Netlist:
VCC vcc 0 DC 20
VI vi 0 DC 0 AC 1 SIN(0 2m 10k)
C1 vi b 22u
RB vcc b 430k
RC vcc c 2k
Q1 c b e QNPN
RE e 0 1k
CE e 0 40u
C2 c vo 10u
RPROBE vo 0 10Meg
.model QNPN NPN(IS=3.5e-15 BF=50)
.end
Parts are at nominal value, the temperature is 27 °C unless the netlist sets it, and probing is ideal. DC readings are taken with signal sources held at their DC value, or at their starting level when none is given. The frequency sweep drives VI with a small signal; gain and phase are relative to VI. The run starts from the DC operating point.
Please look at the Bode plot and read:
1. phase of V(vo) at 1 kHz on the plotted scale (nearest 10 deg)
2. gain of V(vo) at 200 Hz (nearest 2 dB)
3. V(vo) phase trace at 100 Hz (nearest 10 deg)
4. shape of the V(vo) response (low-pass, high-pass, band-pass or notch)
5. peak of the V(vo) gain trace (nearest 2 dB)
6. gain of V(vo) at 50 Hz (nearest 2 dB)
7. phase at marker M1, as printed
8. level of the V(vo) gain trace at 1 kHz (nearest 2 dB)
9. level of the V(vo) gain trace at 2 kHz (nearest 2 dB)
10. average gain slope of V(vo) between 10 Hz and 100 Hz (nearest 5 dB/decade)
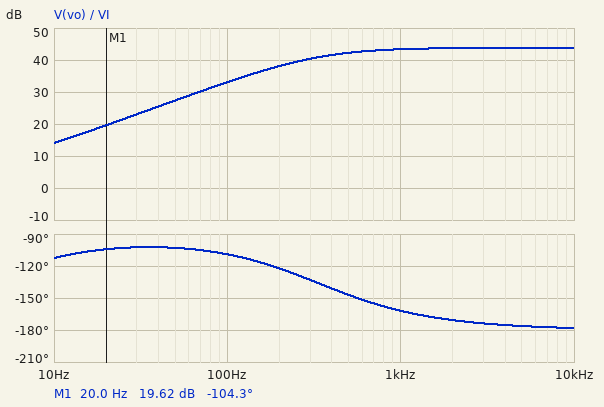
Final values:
-160 deg
38 dB
-110 deg
high-pass
44 dB
28 dB
-104.3 deg
44 dB
44 dB
20 dB/decade
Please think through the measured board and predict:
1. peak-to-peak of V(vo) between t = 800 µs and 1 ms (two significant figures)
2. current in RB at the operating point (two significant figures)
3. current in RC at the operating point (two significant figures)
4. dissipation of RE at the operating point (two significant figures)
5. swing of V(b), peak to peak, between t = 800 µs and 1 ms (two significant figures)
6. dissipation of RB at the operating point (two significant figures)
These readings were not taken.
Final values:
620 mV
40 µA
2.0 mA
4.2 mW
4.0 mV
690 µW
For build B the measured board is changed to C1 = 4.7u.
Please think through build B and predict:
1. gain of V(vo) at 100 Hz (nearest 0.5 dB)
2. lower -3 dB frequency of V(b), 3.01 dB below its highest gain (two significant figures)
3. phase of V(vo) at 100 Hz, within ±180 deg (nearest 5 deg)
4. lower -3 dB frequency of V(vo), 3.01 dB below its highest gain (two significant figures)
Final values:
32.0 dB
910 mHz
-105 deg
370 Hz
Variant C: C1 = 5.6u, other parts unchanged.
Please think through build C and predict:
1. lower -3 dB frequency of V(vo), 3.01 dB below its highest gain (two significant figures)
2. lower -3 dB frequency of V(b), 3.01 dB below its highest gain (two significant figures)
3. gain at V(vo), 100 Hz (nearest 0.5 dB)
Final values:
360 Hz
730 mHz
32.5 dB
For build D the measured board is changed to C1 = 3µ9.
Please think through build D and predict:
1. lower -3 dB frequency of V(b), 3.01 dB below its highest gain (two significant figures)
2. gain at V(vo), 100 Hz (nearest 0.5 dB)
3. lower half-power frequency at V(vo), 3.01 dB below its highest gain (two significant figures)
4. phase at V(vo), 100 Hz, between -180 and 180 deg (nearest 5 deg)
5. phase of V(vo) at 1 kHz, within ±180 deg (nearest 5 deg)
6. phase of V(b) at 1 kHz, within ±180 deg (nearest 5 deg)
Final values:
1.2 Hz
32.0 dB
380 Hz
-105 deg
-160 deg
5 deg
